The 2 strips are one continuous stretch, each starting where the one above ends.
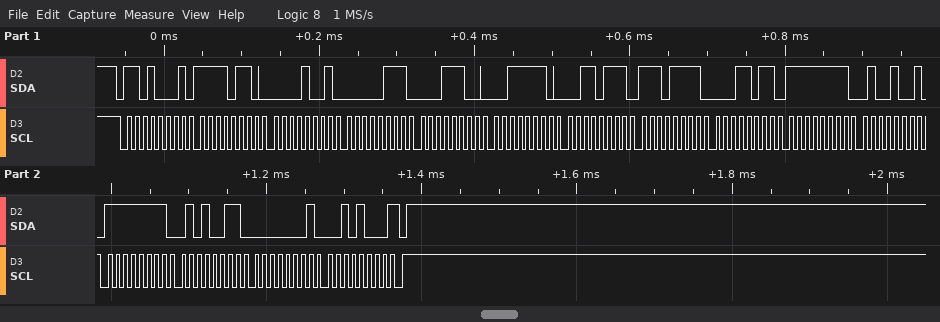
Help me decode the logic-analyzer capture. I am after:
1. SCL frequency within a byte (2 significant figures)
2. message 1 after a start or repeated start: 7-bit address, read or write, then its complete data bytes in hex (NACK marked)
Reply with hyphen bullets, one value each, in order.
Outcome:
- 100 kHz
- 0x68 read: F6 09 07 1C 3E 37 EF 1B FF 49 FF 53 01 28 NACK
